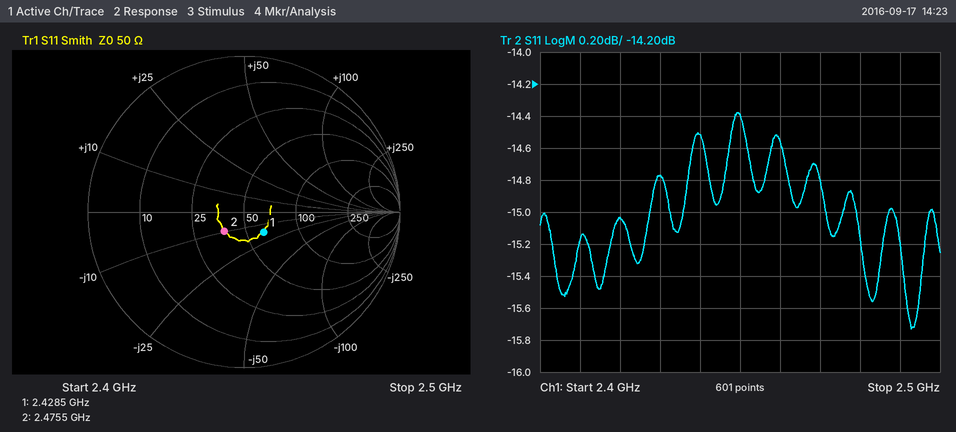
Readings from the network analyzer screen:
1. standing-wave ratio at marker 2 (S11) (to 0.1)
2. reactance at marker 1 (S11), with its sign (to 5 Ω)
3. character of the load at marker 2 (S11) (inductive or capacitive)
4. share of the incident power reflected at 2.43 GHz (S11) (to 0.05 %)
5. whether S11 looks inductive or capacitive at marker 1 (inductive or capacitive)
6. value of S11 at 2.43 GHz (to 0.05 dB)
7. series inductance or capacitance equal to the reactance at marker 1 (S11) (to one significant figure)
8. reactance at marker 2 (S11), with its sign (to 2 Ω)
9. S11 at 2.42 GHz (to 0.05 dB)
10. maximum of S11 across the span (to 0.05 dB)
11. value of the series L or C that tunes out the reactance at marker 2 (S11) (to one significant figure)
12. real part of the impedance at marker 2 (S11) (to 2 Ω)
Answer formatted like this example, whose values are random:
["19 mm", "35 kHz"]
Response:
["1.4", "-15 Ω", "capacitive", "3.35 %", "capacitive", "-14.75 dB", "4 pF", "-10 Ω", "-15.05 dB", "-14.40 dB", "600 pH", "38 Ω"]
